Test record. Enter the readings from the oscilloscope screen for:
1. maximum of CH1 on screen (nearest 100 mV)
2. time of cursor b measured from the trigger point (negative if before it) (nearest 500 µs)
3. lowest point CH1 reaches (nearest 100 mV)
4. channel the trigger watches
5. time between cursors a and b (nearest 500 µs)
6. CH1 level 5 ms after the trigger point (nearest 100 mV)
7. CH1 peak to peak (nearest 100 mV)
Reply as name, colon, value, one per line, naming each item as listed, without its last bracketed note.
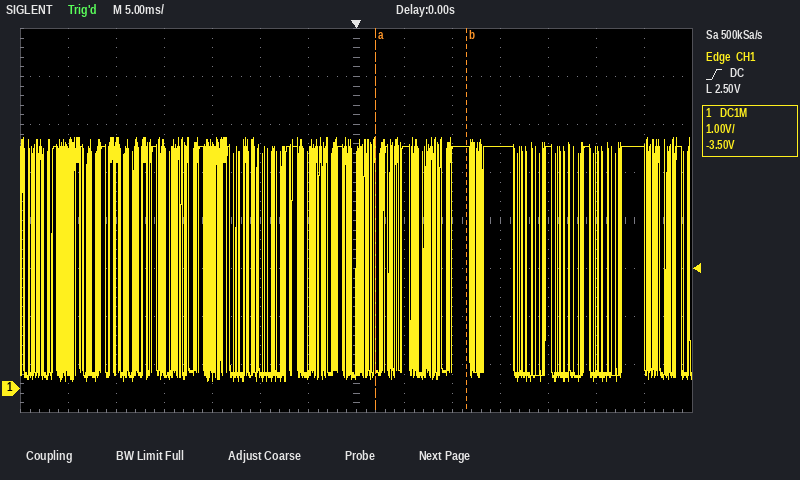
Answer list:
maximum of CH1 on screen: 5.2 V
time of cursor b measured from the trigger point (negative if before it): +11.5 ms
lowest point CH1 reaches: 100 mV
channel the trigger watches: CH1
time between cursors a and b: 9.5 ms
CH1 level 5 ms after the trigger point: 5.0 V
CH1 peak to peak: 5.1 V
